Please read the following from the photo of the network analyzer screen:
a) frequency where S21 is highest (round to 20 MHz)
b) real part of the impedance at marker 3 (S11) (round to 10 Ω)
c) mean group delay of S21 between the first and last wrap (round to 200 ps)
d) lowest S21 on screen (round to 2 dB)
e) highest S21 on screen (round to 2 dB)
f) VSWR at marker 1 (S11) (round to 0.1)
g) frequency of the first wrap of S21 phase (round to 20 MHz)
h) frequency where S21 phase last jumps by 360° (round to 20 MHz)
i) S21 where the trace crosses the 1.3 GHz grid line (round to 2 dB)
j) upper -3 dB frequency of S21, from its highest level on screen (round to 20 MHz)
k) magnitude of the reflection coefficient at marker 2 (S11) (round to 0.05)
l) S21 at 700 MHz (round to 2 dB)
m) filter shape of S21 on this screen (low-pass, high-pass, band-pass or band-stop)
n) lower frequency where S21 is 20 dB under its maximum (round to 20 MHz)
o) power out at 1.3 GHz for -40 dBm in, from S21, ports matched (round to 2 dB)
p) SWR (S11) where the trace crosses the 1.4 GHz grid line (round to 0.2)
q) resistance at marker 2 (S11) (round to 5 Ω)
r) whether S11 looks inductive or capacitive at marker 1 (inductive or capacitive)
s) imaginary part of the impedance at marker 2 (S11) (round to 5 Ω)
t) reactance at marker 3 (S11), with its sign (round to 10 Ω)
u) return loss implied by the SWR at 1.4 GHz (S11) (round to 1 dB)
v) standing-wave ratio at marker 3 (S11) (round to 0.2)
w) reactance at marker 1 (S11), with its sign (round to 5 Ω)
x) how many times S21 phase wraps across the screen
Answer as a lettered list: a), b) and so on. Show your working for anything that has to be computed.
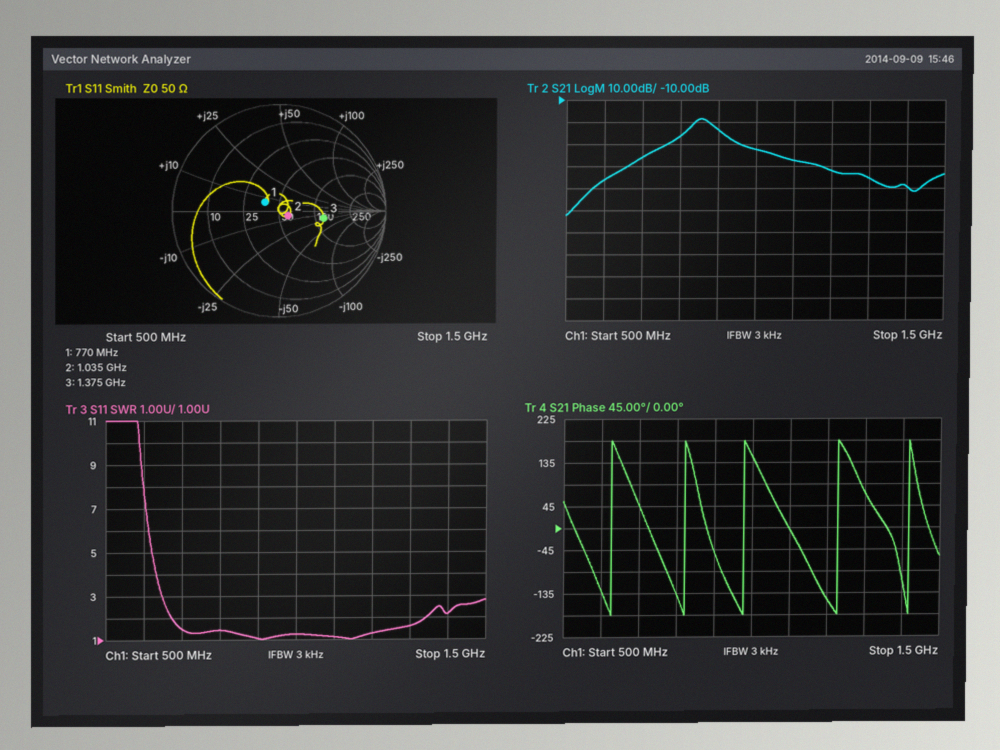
a) 860 MHz
b) 120 Ω
c) 4 cycles / (1.42 GHz − 620 MHz) ≈ 5.0 ns
d) -62 dB
e) -18 dB
f) 1.4
g) 620 MHz
h) 1.42 GHz
i) -46 dB
j) 880 MHz
k) 0.10
l) -36 dB
m) band-pass
n) 680 MHz
o) -40 dBm + (-46 dB) = -86 dBm
p) 2.2
q) 60 Ω
r) inductive
s) -5 Ω
t) -20 Ω
u) −20 log10((2.2 − 1)/(2.2 + 1)) ≈ 9 dB
v) 2.4
w) +5 Ω
x) 5
